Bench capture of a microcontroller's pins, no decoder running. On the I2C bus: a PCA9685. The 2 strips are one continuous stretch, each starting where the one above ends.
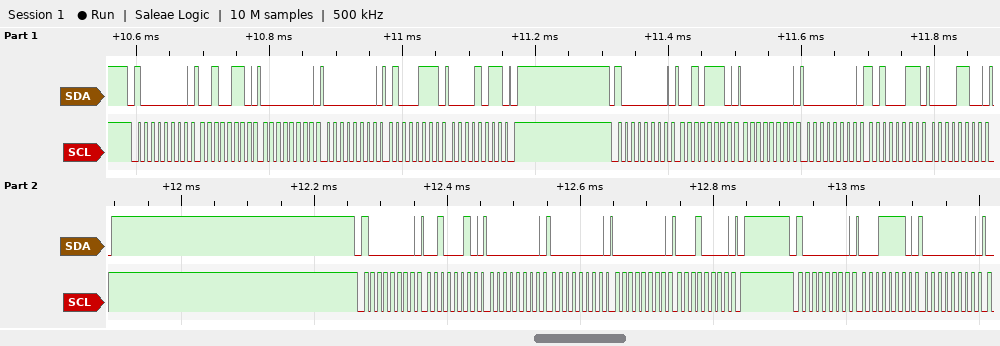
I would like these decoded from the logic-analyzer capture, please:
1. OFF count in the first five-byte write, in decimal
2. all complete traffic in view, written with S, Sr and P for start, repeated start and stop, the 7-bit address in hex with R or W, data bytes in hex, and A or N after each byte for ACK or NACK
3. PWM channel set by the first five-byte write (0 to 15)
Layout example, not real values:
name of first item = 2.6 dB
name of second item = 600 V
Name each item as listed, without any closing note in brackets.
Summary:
OFF count in the first five-byte write, in decimal = 2887
all complete traffic in view, written with S, Sr and P for start, repeated start and stop, the 7-bit address in hex with R or W, data bytes in hex, and A or N after each byte for ACK or NACK = S 40W A 26 A 00 A 00 A 47 A 0B A P S 40W A 2E A 00 A 00 A A3 A 0C A P S 40W A 22 A 00 A 00 A 00 A 10 A P S 40W A 1E A 00 A
PWM channel set by the first five-byte write = 8
